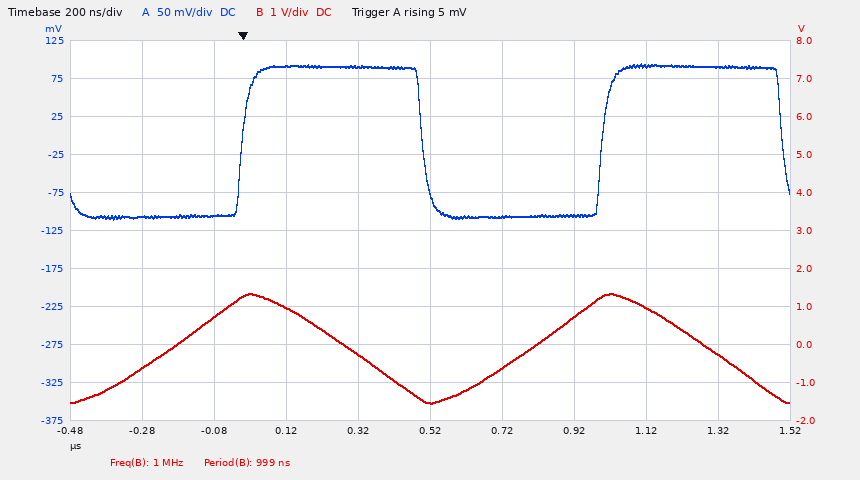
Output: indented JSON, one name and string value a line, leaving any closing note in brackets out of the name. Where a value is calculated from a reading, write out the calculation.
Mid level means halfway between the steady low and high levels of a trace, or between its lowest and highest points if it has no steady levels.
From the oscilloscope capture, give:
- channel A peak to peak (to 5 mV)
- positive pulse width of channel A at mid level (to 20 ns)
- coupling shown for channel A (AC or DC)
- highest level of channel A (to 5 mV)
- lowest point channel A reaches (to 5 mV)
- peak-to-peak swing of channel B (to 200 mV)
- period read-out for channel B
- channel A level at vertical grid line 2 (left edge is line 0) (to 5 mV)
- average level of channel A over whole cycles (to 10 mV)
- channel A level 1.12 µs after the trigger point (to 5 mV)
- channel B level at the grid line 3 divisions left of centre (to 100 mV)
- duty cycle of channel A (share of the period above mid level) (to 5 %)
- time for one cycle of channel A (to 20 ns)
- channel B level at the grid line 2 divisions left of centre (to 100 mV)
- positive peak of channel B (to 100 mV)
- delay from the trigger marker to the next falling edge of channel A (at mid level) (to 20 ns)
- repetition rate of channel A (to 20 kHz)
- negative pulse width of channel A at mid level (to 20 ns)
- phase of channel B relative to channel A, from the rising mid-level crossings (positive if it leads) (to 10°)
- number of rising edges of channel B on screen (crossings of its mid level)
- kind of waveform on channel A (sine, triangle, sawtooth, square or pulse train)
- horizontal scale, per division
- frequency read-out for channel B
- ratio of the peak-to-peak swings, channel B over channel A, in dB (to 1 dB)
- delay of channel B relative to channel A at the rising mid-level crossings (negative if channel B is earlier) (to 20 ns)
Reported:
{
  "channel A peak to peak": "95 mV − (-110 mV) = 205 mV",
  "positive pulse width of channel A at mid level": "500 ns",
  "coupling shown for channel A": "DC",
  "highest level of channel A": "95 mV",
  "lowest point channel A reaches": "-110 mV",
  "peak-to-peak swing of channel B": "2.8 V",
  "period read-out for channel B": "999 ns",
  "channel A level at vertical grid line 2 (left edge is line 0)": "-105 mV",
  "average level of channel A over whole cycles": "-110 mV + 0.5 × (95 mV − (-110 mV)) ≈ -7.50 mV, so -10 mV to the nearest 10 mV",
  "channel A level 1.12 µs after the trigger point": "90 mV",
  "channel B level at the grid line 3 divisions left of centre": "700 mV",
  "duty cycle of channel A (share of the period above mid level)": "500 ns / 1.00 µs ≈ 50 %",
  "time for one cycle of channel A": "1.00 µs",
  "channel B level at the grid line 2 divisions left of centre": "1.0 V",
  "positive peak of channel B": "1.3 V",
  "delay from the trigger marker to the next falling edge of channel A (at mid level)": "500 ns",
  "repetition rate of channel A": "1 / 1.00 µs ≈ 1.00 MHz",
  "negative pulse width of channel A at mid level": "500 ns",
  "phase of channel B relative to channel A, from the rising mid-level crossings (positive if it leads)": "−360° × (-200 ns) / 1.00 µs ≈ +72.0°, so +70° to the nearest 10°",
  "number of rising edges of channel B on screen": "2",
  "kind of waveform on channel A": "square",
  "horizontal scale, per division": "200 ns",
  "frequency read-out for channel B": "1 MHz",
  "ratio of the peak-to-peak swings, channel B over channel A, in dB": "20 log10(2.8 V / 205 mV) ≈ 23 dB",
  "delay of channel B relative to channel A at the rising mid-level crossings (negative if channel B is earlier)": "-200 ns"
}
